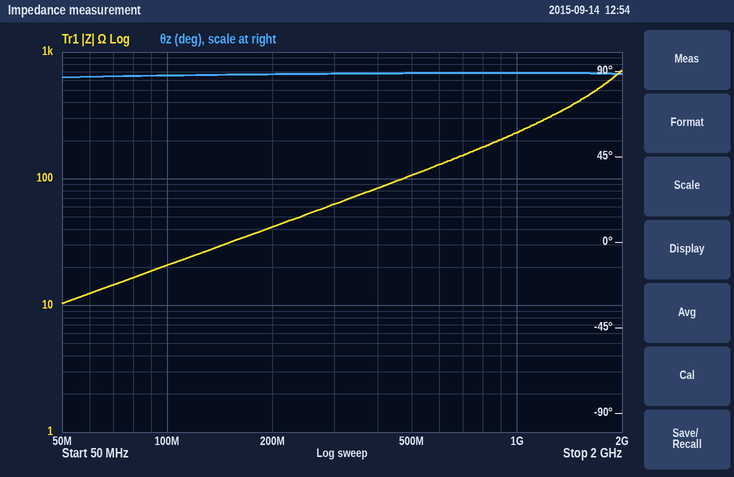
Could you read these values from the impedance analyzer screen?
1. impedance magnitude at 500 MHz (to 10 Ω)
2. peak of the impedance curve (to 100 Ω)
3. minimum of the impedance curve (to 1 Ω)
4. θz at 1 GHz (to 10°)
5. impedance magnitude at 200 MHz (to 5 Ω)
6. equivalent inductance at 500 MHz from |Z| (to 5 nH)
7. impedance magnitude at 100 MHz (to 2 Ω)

110 Ω
700 Ω
10 Ω
90°
40 Ω
35 nH
20 Ω
